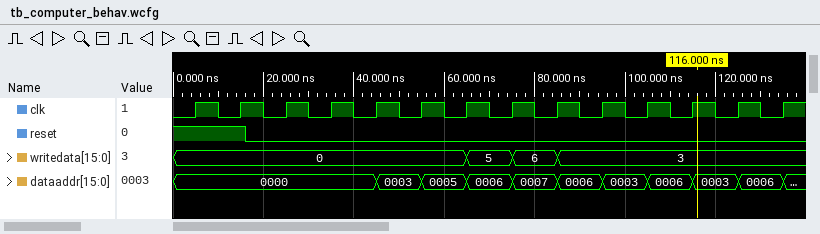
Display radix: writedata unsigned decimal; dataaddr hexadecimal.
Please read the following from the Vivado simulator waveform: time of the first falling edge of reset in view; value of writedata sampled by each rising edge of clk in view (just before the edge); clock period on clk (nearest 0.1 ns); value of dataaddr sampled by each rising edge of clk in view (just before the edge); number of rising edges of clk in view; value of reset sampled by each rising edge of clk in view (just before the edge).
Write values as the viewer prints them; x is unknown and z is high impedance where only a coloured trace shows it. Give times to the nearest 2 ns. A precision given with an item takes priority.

16 ns
0, 0, 0, 0, 0, 0, 0, 5, 6, 3, 3, 3, 3, 3
10 ns
0000, 0000, 0000, 0000, 0000, 0003, 0005, 0006, 0007, 0006, 0003, 0006, 0003, 0006
14
1 1 0 0 0 0 0 0 0 0 0 0 0 0
